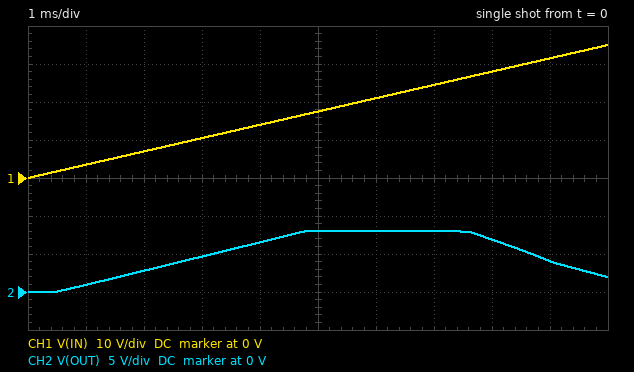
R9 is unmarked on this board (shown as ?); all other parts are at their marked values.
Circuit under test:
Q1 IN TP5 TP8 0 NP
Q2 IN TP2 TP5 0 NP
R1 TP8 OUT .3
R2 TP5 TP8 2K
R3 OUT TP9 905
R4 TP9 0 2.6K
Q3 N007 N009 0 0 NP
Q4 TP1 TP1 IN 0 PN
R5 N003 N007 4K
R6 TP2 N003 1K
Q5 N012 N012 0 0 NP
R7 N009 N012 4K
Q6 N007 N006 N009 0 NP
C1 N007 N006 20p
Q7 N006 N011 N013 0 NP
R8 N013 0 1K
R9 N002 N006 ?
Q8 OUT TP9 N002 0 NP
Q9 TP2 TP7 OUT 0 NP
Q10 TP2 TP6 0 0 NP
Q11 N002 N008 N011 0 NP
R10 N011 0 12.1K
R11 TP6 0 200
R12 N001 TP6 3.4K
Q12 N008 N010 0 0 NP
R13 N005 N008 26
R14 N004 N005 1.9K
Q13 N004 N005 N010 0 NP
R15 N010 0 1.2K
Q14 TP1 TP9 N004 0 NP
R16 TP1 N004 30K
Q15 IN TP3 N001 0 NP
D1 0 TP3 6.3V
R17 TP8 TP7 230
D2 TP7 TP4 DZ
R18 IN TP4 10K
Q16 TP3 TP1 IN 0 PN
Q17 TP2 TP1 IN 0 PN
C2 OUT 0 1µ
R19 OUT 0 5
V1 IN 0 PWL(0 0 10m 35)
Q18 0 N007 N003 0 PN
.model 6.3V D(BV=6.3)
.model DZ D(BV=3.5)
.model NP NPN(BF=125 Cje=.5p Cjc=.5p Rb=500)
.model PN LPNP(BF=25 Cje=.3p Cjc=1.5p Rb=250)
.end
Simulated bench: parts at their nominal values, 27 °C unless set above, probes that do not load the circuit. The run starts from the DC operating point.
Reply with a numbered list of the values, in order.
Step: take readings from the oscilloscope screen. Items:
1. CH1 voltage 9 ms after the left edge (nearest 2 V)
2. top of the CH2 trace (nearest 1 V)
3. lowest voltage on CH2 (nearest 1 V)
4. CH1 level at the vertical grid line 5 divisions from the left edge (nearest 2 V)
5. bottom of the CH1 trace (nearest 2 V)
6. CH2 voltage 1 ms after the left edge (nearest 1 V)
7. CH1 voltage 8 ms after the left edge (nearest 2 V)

1. 32 V
2. 8 V
3. 0 V
4. 18 V
5. 0 V
6. 1 V
7. 28 V
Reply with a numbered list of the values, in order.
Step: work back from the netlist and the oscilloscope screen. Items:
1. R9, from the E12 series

1. 39 kΩ
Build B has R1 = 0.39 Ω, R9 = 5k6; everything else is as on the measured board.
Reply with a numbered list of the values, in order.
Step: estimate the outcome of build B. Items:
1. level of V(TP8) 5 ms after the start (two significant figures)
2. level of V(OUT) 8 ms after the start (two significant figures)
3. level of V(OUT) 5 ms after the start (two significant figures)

1. 3.7 V
2. 3.5 V
3. 3.4 V
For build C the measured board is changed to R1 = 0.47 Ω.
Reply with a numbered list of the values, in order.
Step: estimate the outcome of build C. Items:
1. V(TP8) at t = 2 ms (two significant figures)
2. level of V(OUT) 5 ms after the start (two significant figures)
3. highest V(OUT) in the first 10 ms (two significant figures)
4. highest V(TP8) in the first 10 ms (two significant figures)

1. 3.0 V
2. 7.0 V
3. 7.5 V
4. 8.2 V
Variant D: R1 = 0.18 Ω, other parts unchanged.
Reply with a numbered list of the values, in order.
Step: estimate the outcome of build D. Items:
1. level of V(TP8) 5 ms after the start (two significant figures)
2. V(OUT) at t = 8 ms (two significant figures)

1. 8.3 V
2. 8.0 V
